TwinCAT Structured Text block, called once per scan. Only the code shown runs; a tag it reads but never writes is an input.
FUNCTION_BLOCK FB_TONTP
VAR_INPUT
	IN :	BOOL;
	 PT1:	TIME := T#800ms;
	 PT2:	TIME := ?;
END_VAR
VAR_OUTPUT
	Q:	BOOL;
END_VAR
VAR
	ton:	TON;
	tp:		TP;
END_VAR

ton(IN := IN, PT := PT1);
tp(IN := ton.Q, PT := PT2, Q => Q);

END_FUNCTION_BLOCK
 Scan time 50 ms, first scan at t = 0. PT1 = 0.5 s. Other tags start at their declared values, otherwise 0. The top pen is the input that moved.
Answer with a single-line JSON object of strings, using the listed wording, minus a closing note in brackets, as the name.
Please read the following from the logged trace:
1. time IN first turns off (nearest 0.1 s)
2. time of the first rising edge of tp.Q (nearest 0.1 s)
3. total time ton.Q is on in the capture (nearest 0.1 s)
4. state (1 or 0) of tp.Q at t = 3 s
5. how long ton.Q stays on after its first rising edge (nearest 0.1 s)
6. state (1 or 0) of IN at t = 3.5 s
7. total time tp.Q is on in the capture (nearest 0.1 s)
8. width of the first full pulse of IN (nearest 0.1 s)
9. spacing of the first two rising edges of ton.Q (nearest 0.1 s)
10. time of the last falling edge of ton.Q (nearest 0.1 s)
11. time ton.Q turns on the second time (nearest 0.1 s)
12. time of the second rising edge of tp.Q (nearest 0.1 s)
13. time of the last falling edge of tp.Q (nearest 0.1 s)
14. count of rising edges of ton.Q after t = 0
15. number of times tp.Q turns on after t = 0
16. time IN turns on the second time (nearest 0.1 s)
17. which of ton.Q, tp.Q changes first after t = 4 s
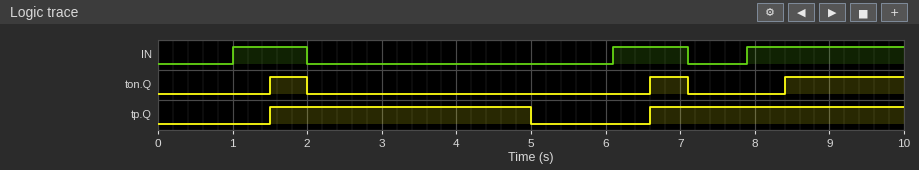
{"time IN first turns off": "2.0 s", "time of the first rising edge of tp.Q": "1.5 s", "total time ton.Q is on in the capture": "2.6 s", "state (1 or 0) of tp.Q at t = 3 s": "1", "how long ton.Q stays on after its first rising edge": "0.5 s", "state (1 or 0) of IN at t = 3.5 s": "0", "total time tp.Q is on in the capture": "6.9 s", "width of the first full pulse of IN": "1.0 s", "spacing of the first two rising edges of ton.Q": "5.1 s", "time of the last falling edge of ton.Q": "7.1 s", "time ton.Q turns on the second time": "6.6 s", "time of the second rising edge of tp.Q": "6.6 s", "time of the last falling edge of tp.Q": "5.0 s", "count of rising edges of ton.Q after t = 0": "3", "number of times tp.Q turns on after t = 0": "2", "time IN turns on the second time": "6.1 s", "which of ton.Q, tp.Q changes first after t = 4 s": "tp.Q"}
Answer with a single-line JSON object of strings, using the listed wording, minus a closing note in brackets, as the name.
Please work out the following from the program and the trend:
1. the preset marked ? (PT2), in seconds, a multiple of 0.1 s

{"the preset marked ? (PT2), in seconds, a multiple of 0.1 s": "3.5 s"}
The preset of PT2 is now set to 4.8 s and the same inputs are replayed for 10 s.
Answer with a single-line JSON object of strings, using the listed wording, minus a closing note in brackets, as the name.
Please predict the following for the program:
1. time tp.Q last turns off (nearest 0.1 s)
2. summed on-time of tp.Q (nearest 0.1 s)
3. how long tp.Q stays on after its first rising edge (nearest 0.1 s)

{"time tp.Q last turns off": "6.3 s", "summed on-time of tp.Q": "8.2 s", "how long tp.Q stays on after its first rising edge": "4.8 s"}
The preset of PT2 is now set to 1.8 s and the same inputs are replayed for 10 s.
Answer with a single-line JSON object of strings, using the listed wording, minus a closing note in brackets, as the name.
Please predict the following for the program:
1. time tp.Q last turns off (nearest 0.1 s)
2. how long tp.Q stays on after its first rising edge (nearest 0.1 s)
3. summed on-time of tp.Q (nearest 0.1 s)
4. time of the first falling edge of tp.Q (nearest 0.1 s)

{"time tp.Q last turns off": "8.4 s", "how long tp.Q stays on after its first rising edge": "1.8 s", "summed on-time of tp.Q": "3.6 s", "time of the first falling edge of tp.Q": "3.3 s"}
